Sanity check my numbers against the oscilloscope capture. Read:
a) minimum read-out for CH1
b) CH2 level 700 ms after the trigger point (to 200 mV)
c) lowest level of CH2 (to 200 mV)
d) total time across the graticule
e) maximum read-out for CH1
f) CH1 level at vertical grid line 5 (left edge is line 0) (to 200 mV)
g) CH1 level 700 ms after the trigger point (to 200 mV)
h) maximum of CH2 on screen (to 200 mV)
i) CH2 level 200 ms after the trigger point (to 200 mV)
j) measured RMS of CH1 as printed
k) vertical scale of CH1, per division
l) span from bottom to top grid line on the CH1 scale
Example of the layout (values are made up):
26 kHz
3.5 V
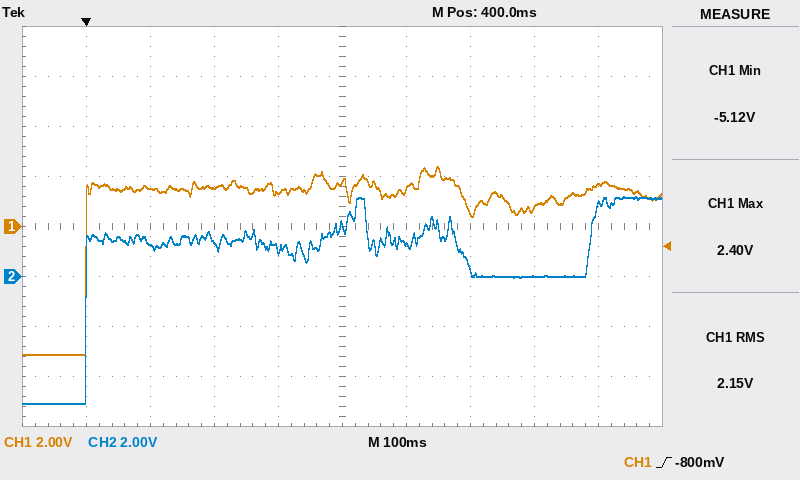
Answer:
-5.12 V
0.0 V
-5.0 V
1 s
2.40 V
1.8 V
800 mV
3.2 V
1.4 V
2.15 V
2 V
16 V
